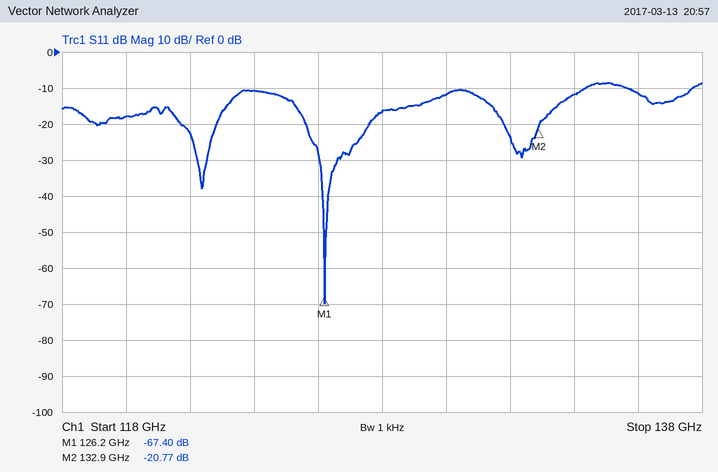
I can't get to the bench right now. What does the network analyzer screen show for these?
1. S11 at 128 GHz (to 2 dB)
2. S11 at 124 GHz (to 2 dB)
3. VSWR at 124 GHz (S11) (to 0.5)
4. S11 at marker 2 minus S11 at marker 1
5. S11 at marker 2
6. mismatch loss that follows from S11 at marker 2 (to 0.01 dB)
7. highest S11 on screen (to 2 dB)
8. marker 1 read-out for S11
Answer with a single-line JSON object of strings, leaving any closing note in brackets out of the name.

{"S11 at 128 GHz": "-16 dB", "S11 at 124 GHz": "-10 dB", "VSWR at 124 GHz (S11)": "2.0", "S11 at marker 2 minus S11 at marker 1": "46.63 dB", "S11 at marker 2": "-20.77 dB", "mismatch loss that follows from S11 at marker 2": "0.04 dB", "highest S11 on screen": "-8 dB", "marker 1 read-out for S11": "-67.40 dB"}
